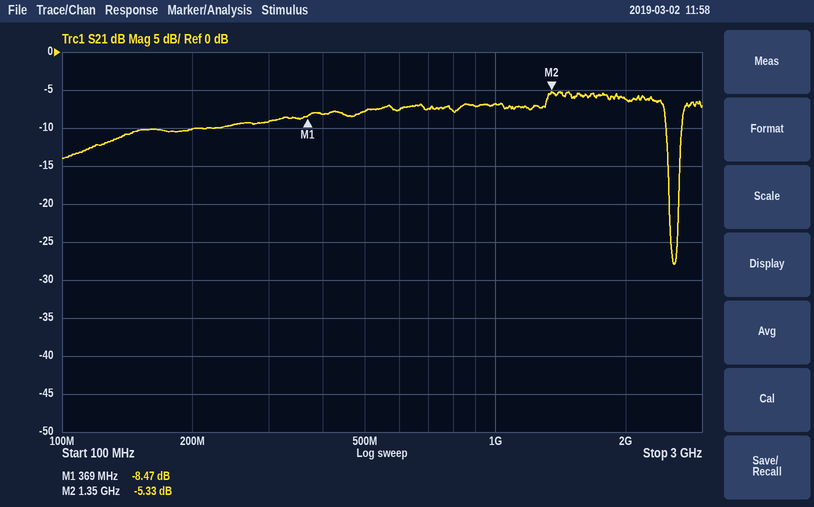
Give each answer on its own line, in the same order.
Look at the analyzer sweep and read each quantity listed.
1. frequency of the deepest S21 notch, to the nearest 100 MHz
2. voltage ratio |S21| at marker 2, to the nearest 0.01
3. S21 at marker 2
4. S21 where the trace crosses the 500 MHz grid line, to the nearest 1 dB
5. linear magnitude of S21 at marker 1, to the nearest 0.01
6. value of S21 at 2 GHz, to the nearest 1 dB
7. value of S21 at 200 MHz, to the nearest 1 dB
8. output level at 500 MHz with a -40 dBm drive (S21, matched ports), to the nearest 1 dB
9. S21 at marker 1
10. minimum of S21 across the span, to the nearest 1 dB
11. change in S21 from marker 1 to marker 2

2.6 GHz
0.54
-5.33 dB
-8 dB
0.38
-6 dB
-10 dB
-48 dBm
-8.47 dB
-28 dB
3.14 dB
